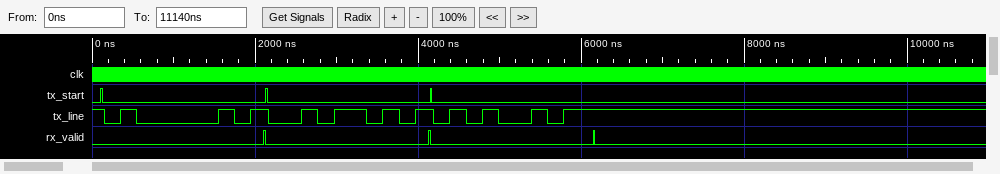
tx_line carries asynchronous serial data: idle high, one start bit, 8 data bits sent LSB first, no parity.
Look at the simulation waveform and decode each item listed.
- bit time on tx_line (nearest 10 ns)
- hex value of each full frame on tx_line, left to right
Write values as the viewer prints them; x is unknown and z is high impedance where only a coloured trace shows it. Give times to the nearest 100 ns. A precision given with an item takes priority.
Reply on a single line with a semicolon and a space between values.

200 ns; 41, 5A, A5
